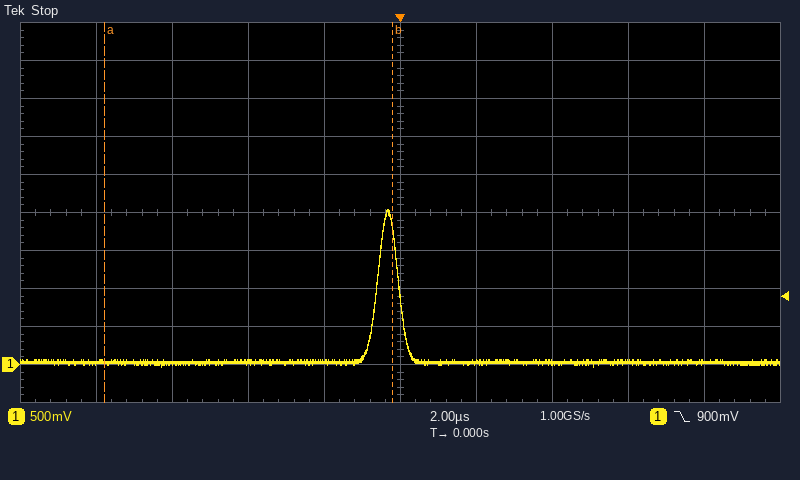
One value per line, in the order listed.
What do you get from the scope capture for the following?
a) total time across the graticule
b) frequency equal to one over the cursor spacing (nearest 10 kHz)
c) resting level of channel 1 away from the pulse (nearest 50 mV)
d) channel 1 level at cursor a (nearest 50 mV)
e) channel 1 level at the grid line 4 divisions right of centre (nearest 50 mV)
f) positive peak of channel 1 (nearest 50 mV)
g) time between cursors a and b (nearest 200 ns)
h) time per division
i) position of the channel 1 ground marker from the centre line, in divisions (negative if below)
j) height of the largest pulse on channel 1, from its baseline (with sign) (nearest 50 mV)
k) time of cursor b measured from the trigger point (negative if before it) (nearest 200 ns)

20 µs
130 kHz
50 mV
50 mV
50 mV
2.05 V
7.6 µs
2 µs
-4.0 div
+2.00 V
-200 ns
